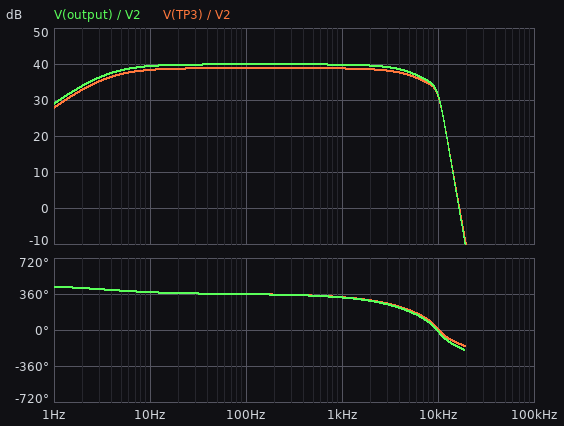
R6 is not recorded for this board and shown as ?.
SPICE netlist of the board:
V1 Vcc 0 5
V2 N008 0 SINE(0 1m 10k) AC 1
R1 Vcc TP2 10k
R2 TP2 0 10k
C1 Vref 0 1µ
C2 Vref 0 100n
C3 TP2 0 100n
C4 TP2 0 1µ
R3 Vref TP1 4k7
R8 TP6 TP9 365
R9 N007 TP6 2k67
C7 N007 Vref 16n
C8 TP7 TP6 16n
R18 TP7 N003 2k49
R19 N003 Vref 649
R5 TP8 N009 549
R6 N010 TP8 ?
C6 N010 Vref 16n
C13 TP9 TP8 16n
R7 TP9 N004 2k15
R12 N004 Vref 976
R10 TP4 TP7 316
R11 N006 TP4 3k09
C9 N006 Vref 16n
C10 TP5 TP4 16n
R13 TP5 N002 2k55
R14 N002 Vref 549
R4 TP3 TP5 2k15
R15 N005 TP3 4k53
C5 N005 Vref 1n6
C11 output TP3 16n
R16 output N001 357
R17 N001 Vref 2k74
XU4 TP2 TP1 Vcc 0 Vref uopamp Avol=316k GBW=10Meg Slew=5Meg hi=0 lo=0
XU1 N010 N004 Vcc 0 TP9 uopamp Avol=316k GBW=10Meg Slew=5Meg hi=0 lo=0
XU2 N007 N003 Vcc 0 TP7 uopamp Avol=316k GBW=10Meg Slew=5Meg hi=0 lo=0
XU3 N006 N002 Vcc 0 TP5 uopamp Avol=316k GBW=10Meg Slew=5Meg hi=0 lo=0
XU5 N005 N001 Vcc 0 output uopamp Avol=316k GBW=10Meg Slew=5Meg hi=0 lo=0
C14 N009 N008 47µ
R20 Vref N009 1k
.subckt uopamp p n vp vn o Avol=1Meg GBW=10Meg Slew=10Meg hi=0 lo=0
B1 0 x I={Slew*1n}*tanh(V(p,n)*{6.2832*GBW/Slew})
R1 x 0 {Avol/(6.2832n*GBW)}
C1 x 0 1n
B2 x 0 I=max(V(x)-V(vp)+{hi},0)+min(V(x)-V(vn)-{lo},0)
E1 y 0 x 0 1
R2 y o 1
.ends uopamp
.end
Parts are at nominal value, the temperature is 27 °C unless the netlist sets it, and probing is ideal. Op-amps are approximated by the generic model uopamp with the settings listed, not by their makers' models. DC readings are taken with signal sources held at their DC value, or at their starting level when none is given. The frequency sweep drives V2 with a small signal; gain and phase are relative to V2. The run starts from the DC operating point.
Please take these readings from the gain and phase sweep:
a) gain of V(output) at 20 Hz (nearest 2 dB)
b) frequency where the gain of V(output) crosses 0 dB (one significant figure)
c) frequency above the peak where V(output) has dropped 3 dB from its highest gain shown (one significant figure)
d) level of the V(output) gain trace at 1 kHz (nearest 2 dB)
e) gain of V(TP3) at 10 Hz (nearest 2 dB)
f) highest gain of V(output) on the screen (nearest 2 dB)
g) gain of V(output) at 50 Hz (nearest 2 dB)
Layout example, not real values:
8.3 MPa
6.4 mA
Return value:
40 dB
20 kHz
6 kHz
40 dB
38 dB
40 dB
40 dB
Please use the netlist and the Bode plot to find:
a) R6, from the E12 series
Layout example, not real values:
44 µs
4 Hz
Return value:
2.7 kΩ
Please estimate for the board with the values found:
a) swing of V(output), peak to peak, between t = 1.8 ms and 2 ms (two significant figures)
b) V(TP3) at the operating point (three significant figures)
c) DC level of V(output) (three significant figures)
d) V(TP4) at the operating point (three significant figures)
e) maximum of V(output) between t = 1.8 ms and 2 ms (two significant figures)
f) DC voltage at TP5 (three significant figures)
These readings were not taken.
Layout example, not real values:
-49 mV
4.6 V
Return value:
75 mV
2.50 V
2.50 V
2.50 V
2.5 V
2.50 V
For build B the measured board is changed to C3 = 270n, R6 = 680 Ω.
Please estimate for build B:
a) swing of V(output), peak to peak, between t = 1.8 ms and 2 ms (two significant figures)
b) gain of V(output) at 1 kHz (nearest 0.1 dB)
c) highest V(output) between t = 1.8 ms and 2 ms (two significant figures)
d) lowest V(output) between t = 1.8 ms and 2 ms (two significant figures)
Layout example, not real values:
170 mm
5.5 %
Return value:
260 mV
39.9 dB
2.6 V
2.4 V
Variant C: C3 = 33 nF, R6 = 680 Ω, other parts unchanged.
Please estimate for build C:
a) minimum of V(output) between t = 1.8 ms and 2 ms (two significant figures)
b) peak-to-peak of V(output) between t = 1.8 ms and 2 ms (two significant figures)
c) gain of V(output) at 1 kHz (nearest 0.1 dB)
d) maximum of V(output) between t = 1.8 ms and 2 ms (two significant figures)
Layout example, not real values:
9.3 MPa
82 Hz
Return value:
2.4 V
260 mV
39.9 dB
2.6 V
